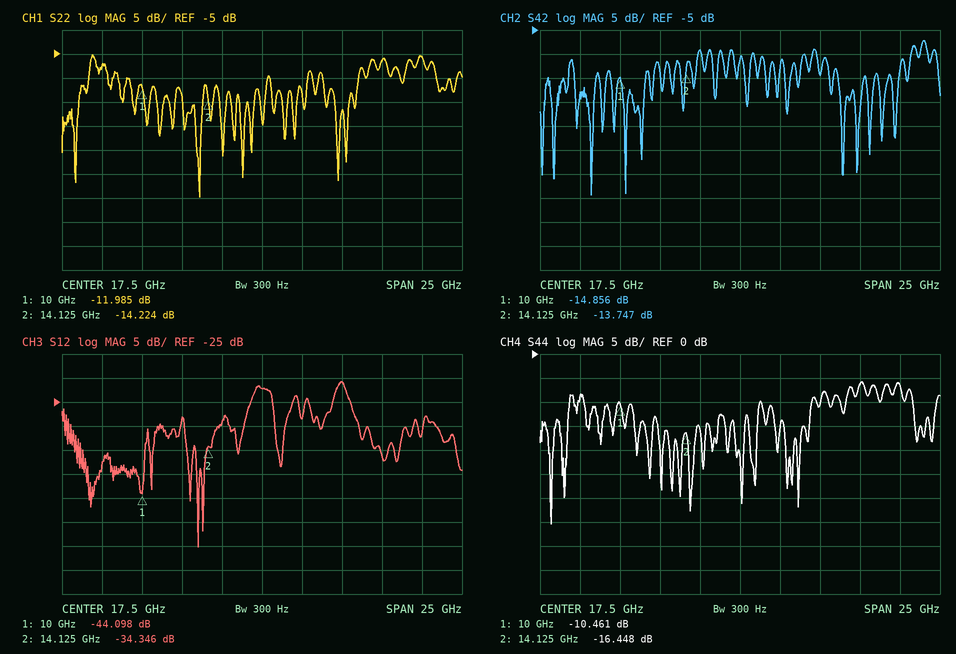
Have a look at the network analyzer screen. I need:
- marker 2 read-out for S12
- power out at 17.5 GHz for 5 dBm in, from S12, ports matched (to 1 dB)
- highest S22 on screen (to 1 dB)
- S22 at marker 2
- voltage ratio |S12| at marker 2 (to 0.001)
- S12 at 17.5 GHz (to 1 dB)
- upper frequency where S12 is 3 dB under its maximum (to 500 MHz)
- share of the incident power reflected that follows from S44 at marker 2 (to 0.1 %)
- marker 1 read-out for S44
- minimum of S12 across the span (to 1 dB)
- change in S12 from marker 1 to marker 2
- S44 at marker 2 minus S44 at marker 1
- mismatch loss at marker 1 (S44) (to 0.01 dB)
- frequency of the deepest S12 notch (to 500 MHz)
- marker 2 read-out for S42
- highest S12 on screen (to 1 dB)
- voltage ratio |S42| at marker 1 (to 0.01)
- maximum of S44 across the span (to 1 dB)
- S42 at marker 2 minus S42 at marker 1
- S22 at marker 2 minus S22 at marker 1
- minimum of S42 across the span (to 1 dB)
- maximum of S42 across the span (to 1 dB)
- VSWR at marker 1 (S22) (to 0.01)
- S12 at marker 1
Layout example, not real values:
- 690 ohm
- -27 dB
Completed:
- -34.346 dB
- -17 dBm
- -5 dB
- -14.224 dB
- 0.019
- -22 dB
- 23.0 GHz
- 2.3 %
- -10.461 dB
- -55 dB
- 9.752 dB
- -5.987 dB
- 0.41 dB
- 13.5 GHz
- -13.747 dB
- -21 dB
- 0.18
- -6 dB
- 1.109 dB
- -2.239 dB
- -39 dB
- -7 dB
- 1.67
- -44.098 dB
